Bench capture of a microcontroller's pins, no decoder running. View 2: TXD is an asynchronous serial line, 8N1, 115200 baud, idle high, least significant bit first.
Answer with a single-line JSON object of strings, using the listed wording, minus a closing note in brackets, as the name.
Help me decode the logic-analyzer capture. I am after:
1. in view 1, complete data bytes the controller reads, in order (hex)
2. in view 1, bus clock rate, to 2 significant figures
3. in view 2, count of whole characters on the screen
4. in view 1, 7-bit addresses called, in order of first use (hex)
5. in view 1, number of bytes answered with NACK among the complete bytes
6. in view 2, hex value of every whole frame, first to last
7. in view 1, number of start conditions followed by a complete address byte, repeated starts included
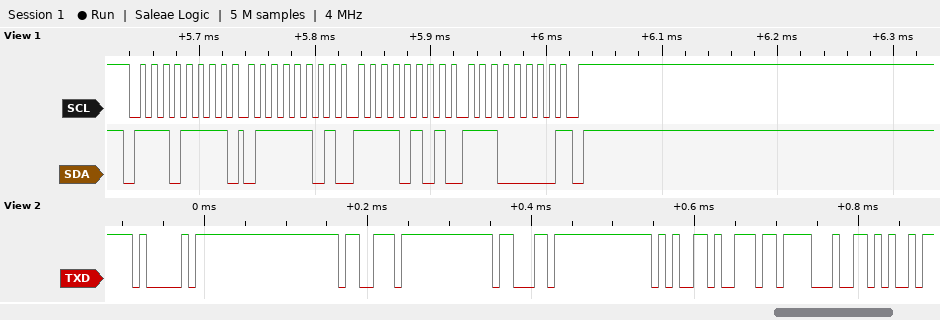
{"in view 1, complete data bytes the controller reads, in order": "7D F5 E0", "in view 1, bus clock rate, to 2 significant figures": "100 kHz", "in view 2, count of whole characters on the screen": "6", "in view 1, 7-bit addresses called, in order of first use": "0x77", "in view 1, number of bytes answered with NACK among the complete bytes": "1", "in view 2, hex value of every whole frame, first to last": "41 73 63 65 6E 64", "in view 1, number of start conditions followed by a complete address byte, repeated starts included": "1"}
